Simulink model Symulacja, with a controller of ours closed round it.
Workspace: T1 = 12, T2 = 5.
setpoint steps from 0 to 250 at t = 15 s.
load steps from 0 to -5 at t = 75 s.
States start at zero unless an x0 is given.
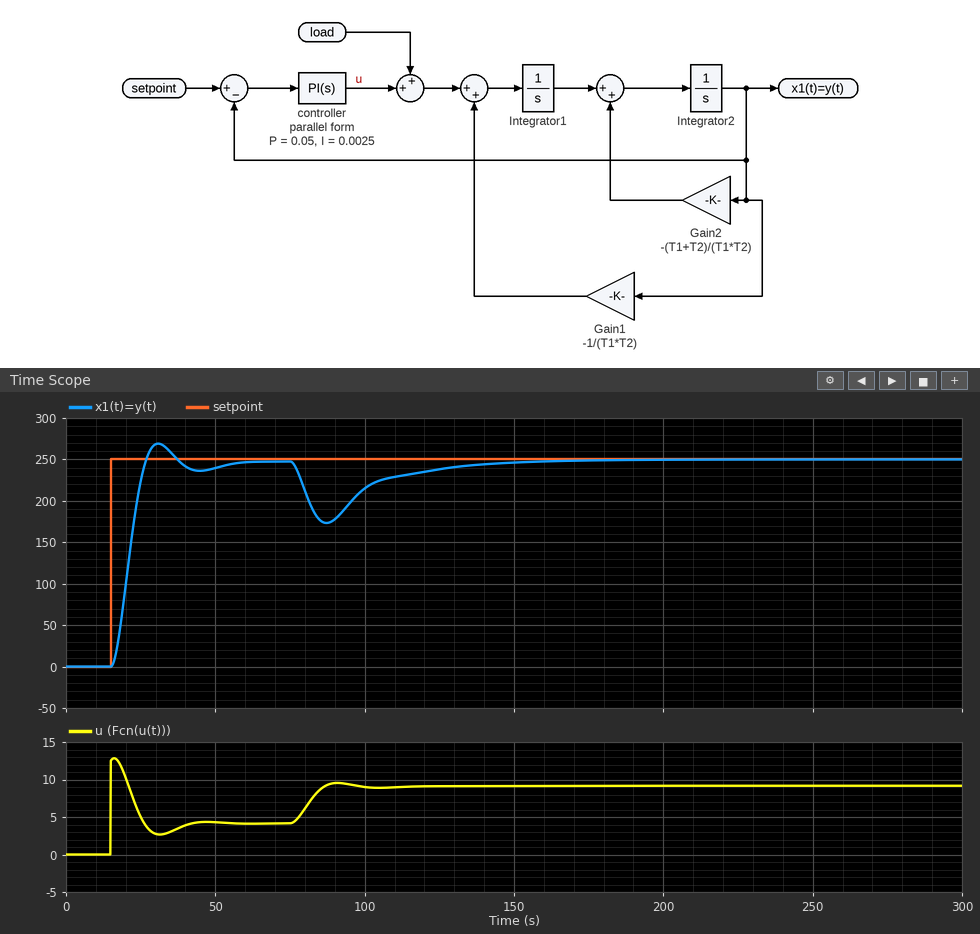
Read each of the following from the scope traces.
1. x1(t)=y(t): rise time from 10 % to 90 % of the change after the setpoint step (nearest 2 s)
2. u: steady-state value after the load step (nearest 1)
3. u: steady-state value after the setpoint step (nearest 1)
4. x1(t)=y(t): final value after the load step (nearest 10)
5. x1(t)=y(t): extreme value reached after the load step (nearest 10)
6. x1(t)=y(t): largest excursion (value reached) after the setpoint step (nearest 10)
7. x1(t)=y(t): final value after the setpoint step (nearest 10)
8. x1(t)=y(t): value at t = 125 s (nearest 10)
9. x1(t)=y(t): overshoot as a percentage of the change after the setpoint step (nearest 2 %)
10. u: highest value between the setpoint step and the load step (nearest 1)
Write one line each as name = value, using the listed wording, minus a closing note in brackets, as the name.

x1(t)=y(t): rise time from 10 % to 90 % of the change after the setpoint step = 8 s
u: steady-state value after the load step = 9
u: steady-state value after the setpoint step = 4
x1(t)=y(t): final value after the load step = 250
x1(t)=y(t): extreme value reached after the load step = 170
x1(t)=y(t): largest excursion (value reached) after the setpoint step = 270
x1(t)=y(t): final value after the setpoint step = 250
x1(t)=y(t): value at t = 125 s = 240
x1(t)=y(t): overshoot as a percentage of the change after the setpoint step = 8 %
u: highest value between the setpoint step and the load step = 13
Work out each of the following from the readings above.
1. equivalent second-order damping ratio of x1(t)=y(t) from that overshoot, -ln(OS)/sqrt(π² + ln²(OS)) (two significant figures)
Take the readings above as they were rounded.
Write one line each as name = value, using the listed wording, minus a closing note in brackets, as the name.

equivalent second-order damping ratio of x1(t)=y(t) from that overshoot, -ln(OS)/sqrt(π² + ln²(OS)) = 0.63
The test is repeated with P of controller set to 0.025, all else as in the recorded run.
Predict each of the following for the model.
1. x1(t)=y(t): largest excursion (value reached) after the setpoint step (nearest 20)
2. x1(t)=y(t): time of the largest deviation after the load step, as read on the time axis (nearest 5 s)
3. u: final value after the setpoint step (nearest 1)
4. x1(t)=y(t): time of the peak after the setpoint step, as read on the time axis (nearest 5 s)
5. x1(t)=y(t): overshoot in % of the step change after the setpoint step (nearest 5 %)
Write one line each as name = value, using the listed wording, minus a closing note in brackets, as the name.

x1(t)=y(t): largest excursion (value reached) after the setpoint step = 280
x1(t)=y(t): time of the largest deviation after the load step, as read on the time axis = 90 s
u: final value after the setpoint step = 4
x1(t)=y(t): time of the peak after the setpoint step, as read on the time axis = 40 s
x1(t)=y(t): overshoot in % of the step change after the setpoint step = 15 %
